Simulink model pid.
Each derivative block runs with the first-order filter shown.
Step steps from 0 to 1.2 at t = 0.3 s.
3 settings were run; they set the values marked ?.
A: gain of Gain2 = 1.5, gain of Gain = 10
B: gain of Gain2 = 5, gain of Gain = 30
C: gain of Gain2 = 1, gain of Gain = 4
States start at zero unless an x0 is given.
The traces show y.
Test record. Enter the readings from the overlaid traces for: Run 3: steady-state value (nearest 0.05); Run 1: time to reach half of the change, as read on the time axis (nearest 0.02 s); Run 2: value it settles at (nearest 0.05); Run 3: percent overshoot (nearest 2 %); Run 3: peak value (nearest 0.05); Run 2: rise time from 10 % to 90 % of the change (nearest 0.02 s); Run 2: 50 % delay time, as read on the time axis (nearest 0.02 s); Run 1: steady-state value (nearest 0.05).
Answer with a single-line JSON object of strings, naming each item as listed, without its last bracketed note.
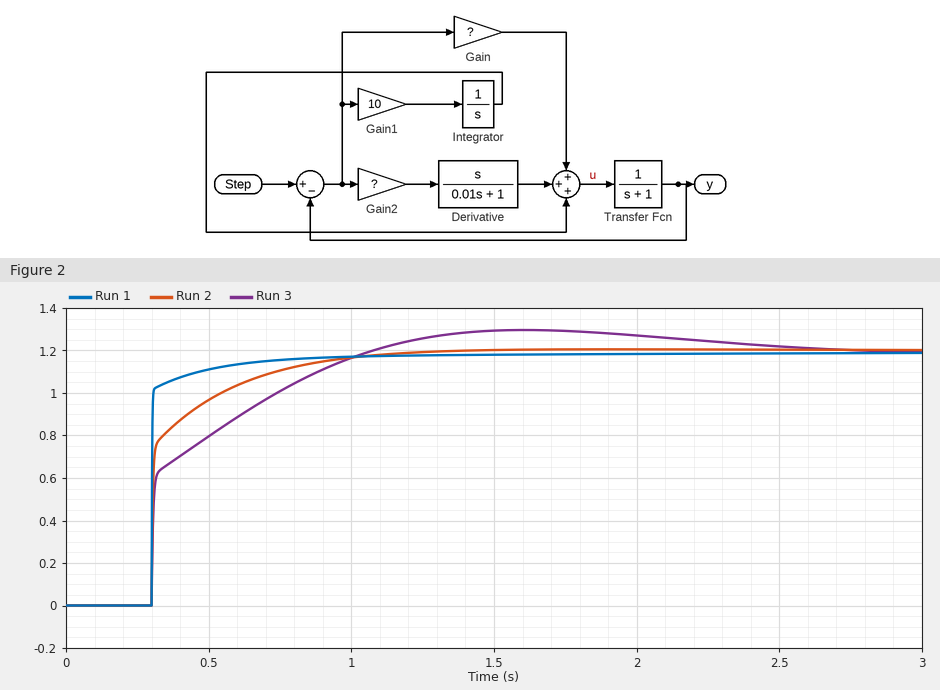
{"Run 3: steady-state value": "1.20", "Run 1: time to reach half of the change, as read on the time axis": "0.30 s", "Run 2: value it settles at": "1.20", "Run 3: percent overshoot": "8 %", "Run 3: peak value": "1.30", "Run 2: rise time from 10 % to 90 % of the change": "0.38 s", "Run 2: 50 % delay time, as read on the time axis": "0.30 s", "Run 1: steady-state value": "1.20"}
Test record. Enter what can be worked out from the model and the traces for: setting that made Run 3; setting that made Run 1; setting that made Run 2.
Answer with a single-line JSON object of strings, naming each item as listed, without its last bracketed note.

{"setting that made Run 3": "C", "setting that made Run 1": "B", "setting that made Run 2": "A"}
